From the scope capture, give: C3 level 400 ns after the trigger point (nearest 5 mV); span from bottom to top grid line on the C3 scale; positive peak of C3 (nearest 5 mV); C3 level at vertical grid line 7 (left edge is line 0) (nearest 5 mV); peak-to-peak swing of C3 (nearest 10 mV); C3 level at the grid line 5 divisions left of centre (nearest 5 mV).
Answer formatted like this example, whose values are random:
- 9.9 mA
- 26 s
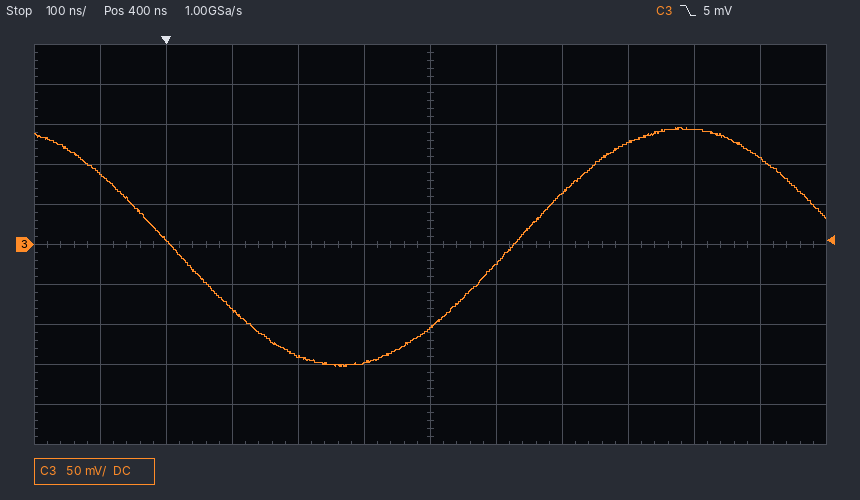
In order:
- -105 mV
- 500 mV
- 145 mV
- -25 mV
- 300 mV
- 90 mV
